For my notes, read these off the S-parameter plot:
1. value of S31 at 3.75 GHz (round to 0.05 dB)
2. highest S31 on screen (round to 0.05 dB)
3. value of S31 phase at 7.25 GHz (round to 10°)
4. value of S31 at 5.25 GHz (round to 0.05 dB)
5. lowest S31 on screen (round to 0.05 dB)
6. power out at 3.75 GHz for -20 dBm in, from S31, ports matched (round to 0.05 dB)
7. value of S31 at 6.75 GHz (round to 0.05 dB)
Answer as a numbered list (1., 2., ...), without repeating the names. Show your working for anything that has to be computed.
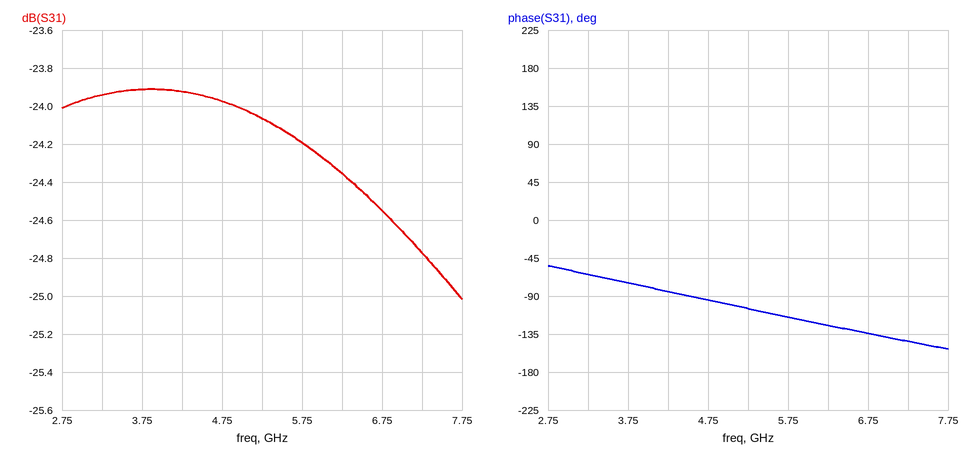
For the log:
1. -23.90 dB
2. -23.90 dB
3. -140°
4. -24.05 dB
5. -25.00 dB
6. -20 dBm + (-23.90 dB) = -43.90 dBm
7. -24.55 dB
